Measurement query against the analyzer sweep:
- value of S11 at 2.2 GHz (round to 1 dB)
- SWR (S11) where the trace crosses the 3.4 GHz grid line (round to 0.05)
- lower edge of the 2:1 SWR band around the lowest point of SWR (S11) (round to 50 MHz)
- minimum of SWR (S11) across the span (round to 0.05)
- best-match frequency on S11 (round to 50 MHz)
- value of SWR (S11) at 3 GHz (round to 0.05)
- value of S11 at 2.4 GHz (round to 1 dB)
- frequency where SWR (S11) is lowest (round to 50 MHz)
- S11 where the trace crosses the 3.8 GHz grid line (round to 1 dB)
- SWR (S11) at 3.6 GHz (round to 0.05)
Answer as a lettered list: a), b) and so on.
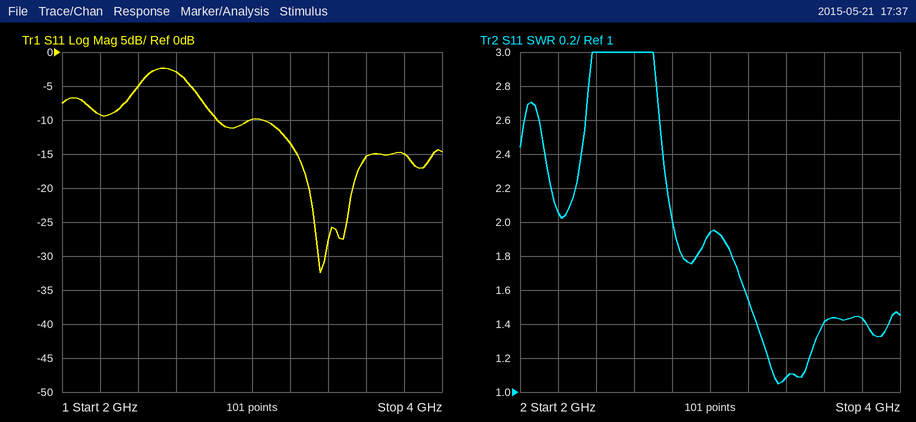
a) -9 dB
b) 1.10
c) 2.80 GHz
d) 1.05
e) 3.35 GHz
f) 1.95
g) -5 dB
h) 3.35 GHz
i) -15 dB
j) 1.40
